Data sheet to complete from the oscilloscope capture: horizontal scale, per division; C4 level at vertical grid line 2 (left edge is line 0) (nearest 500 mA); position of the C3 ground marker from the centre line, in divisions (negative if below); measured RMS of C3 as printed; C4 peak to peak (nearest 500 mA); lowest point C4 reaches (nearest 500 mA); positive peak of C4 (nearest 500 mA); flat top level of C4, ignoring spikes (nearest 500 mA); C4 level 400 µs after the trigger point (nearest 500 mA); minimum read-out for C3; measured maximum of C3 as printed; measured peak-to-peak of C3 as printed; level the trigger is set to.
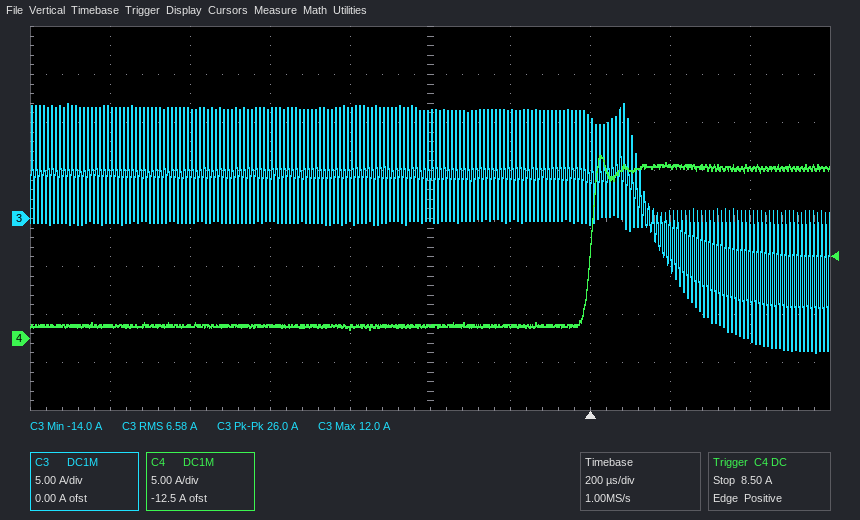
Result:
200 µs
1.5 A
0.0 div
6.58 A
18.0 A
1.0 A
19.0 A
18.0 A
18.0 A
-14.0 A
12.0 A
26.0 A
8.50 A
